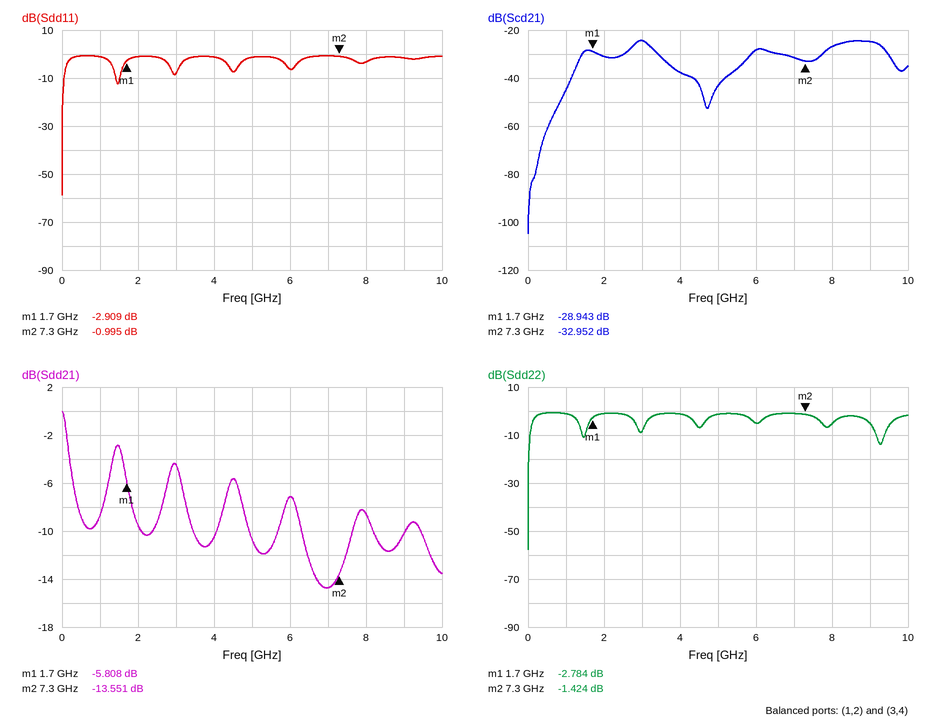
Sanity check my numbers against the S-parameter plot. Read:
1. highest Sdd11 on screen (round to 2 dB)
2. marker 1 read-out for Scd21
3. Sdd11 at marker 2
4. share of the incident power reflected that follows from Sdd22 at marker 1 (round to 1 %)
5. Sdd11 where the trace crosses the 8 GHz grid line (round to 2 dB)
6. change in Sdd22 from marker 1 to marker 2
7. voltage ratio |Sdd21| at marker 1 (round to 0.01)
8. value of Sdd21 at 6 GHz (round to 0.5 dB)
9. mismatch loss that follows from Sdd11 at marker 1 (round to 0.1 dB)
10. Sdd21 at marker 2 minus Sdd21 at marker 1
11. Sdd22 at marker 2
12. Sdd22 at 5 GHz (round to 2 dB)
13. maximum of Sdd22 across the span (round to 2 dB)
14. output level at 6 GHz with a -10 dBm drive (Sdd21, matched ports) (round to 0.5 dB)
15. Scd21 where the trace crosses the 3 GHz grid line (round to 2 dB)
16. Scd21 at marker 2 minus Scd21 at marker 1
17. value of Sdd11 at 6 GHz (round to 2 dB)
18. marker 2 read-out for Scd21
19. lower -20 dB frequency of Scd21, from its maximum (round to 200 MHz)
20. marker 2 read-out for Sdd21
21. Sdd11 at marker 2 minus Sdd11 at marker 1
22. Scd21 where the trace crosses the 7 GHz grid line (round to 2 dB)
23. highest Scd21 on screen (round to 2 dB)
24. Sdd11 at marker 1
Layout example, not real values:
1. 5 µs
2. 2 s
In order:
1. 0 dB
2. -28.943 dB
3. -0.995 dB
4. 53 %
5. -4 dB
6. 1.360 dB
7. 0.51
8. -7.0 dB
9. 3.1 dB
10. -7.743 dB
11. -1.424 dB
12. -2 dB
13. 0 dB
14. -17.0 dBm
15. -24 dB
16. -4.009 dB
17. -6 dB
18. -32.952 dB
19. 1.0 GHz
20. -13.551 dB
21. 1.914 dB
22. -32 dB
23. -24 dB
24. -2.909 dB
